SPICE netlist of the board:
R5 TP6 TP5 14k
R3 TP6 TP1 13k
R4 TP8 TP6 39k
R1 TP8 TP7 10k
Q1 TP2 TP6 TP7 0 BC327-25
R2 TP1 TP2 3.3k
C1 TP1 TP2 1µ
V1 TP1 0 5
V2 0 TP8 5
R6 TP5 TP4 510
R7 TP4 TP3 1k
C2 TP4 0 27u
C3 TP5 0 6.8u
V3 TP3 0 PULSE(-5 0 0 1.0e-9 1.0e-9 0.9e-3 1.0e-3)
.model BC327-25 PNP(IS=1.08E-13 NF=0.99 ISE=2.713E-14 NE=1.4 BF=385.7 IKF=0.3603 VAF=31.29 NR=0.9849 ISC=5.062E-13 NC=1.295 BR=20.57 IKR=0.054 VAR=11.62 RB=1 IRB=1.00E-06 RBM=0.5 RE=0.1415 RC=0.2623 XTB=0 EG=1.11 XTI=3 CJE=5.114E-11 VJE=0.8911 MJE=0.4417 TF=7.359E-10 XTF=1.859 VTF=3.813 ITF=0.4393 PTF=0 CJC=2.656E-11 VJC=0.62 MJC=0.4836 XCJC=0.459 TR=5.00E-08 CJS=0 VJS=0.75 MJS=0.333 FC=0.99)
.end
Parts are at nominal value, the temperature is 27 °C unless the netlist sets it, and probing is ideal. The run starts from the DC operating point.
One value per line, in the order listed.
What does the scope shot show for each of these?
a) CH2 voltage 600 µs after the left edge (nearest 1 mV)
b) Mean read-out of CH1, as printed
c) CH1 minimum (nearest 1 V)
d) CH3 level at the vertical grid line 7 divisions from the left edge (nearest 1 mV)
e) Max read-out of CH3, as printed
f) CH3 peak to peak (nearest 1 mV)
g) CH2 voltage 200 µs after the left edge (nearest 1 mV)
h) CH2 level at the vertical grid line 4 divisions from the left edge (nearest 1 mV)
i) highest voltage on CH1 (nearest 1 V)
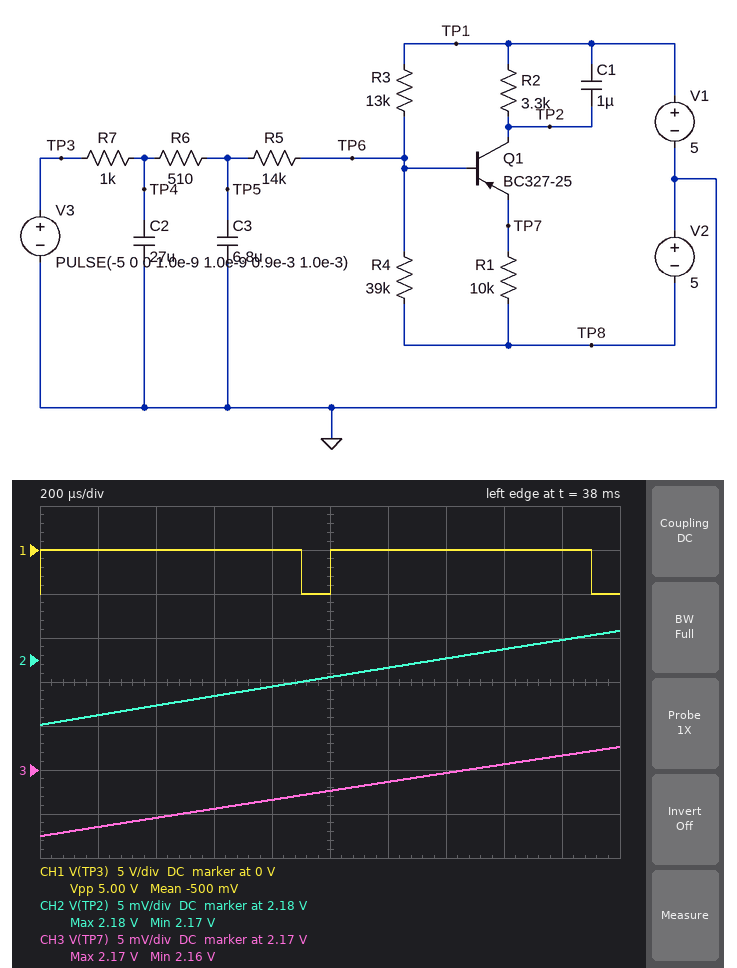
2.176 V
-500 mV
-5 V
2.170 V
2.17 V
10 mV
2.174 V
2.177 V
0 V
